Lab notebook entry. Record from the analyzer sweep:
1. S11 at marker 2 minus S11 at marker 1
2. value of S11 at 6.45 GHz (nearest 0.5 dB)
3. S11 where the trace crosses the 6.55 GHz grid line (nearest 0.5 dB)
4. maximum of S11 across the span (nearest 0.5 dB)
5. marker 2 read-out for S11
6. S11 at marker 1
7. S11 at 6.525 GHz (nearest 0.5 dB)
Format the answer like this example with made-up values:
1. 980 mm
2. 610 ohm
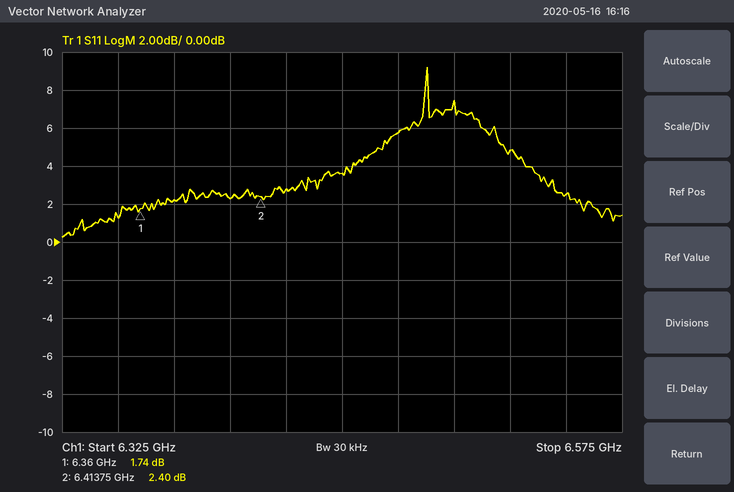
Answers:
1. 0.66 dB
2. 3.5 dB
3. 2.5 dB
4. 9.0 dB
5. 2.40 dB
6. 1.74 dB
7. 5.0 dB
